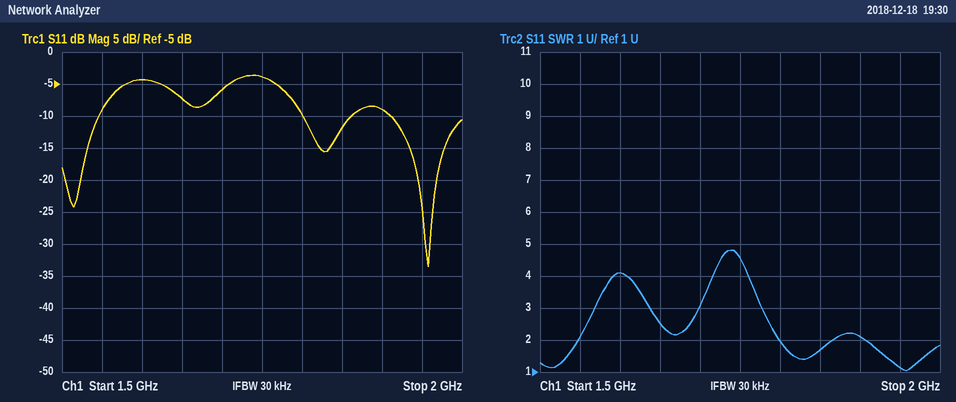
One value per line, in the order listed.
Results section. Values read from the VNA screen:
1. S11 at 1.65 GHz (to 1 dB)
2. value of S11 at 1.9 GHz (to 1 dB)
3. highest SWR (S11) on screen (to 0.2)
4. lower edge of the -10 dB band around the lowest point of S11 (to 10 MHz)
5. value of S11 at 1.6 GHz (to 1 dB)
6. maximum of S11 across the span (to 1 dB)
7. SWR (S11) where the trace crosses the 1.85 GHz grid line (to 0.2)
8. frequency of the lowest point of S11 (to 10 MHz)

-7 dB
-9 dB
4.8
1.91 GHz
-4 dB
-4 dB
1.6
1.96 GHz
